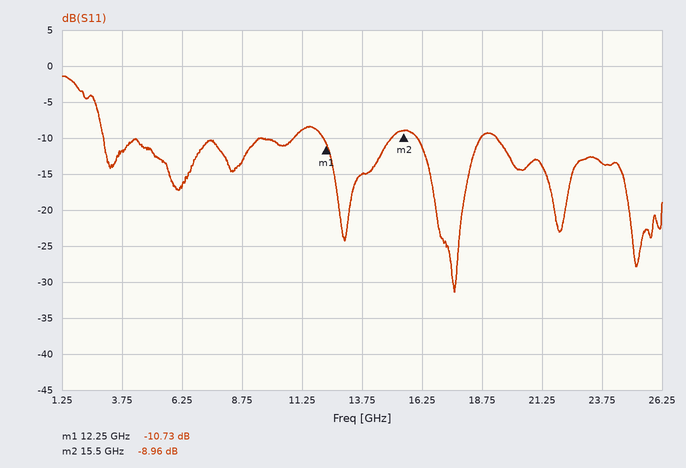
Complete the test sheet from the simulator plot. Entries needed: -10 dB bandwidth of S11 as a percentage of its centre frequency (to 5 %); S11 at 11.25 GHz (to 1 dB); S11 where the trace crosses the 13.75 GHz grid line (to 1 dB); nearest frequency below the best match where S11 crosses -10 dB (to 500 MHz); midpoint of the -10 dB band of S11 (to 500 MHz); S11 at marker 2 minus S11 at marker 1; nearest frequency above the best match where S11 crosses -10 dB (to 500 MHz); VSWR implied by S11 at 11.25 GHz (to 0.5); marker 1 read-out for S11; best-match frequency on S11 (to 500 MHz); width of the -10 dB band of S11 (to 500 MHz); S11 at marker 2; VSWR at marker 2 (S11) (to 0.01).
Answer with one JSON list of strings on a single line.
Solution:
["15 %", "-9 dB", "-15 dB", "16.0 GHz", "17.5 GHz", "1.77 dB", "18.5 GHz", "2.0", "-10.73 dB", "17.5 GHz", "2.5 GHz", "-8.96 dB", "2.11"]
